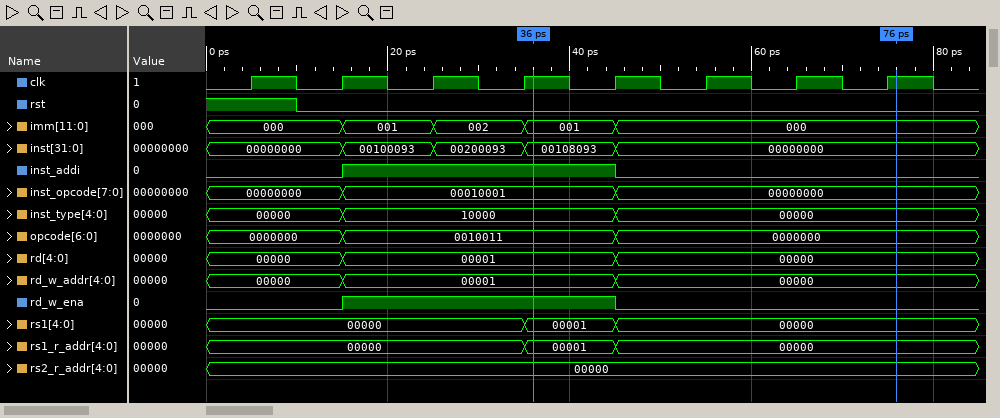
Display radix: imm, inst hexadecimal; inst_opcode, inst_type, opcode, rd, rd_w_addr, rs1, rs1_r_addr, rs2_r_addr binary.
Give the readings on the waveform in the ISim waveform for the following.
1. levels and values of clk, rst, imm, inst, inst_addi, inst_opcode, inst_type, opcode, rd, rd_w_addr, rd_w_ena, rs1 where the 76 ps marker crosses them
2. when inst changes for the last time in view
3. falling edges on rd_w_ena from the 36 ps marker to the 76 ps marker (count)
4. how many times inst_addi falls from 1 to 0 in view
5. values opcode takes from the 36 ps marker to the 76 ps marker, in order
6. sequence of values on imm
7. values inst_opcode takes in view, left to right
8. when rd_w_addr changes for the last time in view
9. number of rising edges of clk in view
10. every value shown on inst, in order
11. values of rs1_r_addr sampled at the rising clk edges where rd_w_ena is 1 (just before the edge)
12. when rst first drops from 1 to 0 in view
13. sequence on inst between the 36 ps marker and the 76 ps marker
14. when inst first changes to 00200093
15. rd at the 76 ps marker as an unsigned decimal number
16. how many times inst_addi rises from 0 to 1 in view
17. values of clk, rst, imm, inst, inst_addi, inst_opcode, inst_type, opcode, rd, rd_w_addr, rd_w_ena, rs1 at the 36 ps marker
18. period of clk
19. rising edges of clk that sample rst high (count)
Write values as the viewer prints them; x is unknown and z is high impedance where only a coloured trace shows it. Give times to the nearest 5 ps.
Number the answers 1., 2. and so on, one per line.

1. clk=1, rst=0, imm=000, inst=00000000, inst_addi=0, inst_opcode=00000000, inst_type=00000, opcode=0000000, rd=00000, rd_w_addr=00000, rd_w_ena=0, rs1=00000
2. 45 ps
3. 1
4. 1
5. 0010011, 0000000
6. 000, 001, 002, 001, 000
7. 00000000, 00010001, 00000000
8. 45 ps
9. 8
10. 00000000, 00100093, 00200093, 00108093, 00000000
11. 00000, 00000, 00001
12. 10 ps
13. 00108093, 00000000
14. 25 ps
15. 0
16. 1
17. clk=1, rst=0, imm=001, inst=00108093, inst_addi=1, inst_opcode=00010001, inst_type=10000, opcode=0010011, rd=00001, rd_w_addr=00001, rd_w_ena=1, rs1=00001
18. 10 ps
19. 1
